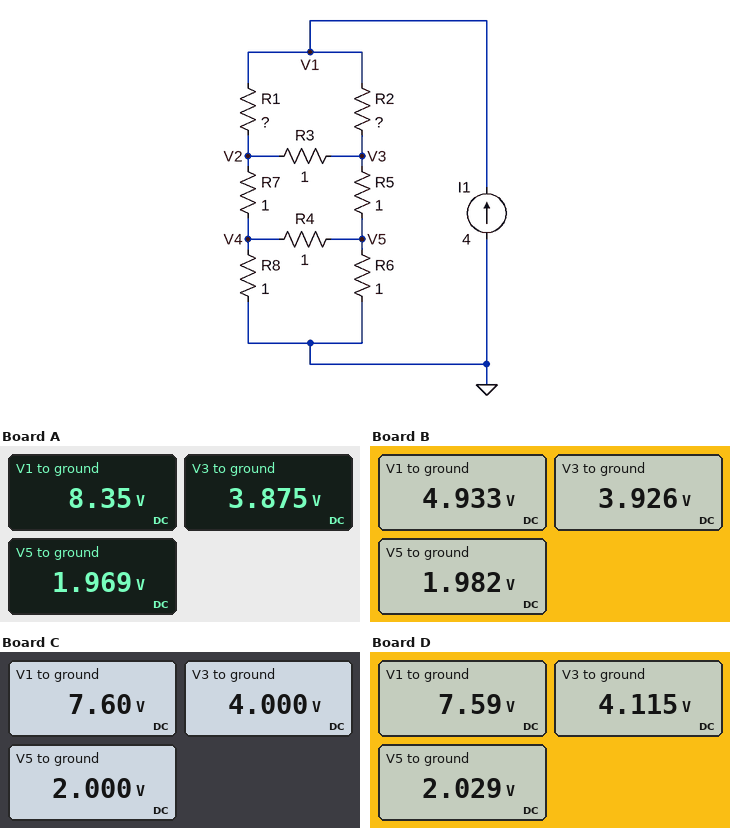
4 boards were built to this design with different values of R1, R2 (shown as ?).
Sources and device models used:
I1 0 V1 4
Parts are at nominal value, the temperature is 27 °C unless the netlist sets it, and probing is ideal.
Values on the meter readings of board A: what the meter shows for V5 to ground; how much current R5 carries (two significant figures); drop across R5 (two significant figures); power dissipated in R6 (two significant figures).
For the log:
1.969 V
1.9 A
1.9 V
3.9 W
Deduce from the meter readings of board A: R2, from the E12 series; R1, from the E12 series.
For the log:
2.7 Ω
1.8 Ω
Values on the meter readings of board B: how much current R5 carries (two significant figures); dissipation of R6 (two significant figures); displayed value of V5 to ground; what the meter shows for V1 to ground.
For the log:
1.9 A
3.9 W
1.982 V
4.933 V
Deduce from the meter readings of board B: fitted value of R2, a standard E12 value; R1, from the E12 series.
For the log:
0.56 Ω
0.39 Ω
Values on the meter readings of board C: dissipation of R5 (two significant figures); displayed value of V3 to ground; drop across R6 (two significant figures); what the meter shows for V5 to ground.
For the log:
4.0 W
4.000 V
2.0 V
2.000 V
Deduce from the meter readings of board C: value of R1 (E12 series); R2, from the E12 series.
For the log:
1.8 Ω
1.8 Ω
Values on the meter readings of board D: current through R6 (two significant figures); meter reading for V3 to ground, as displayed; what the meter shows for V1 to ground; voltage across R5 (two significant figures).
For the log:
2.0 A
4.115 V
7.59 V
2.1 V
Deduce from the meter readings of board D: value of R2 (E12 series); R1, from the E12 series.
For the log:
1.5 Ω
2.2 Ω
